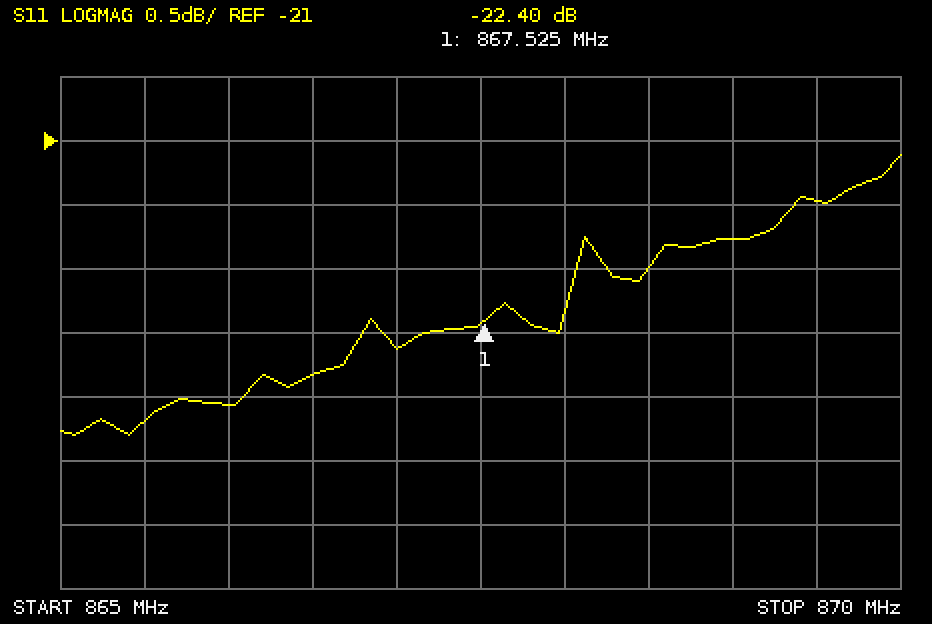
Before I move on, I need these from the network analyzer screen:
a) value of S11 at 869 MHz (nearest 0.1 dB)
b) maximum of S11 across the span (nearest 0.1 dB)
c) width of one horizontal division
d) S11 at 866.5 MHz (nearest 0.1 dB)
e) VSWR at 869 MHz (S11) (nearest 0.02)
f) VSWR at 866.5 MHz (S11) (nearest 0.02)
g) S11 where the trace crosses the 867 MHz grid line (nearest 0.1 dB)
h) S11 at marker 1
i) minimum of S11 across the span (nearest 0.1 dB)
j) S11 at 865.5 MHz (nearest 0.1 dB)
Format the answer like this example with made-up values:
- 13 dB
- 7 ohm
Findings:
- -21.8 dB
- -21.1 dB
- 500 kHz
- -22.8 dB
- 1.18
- 1.16
- -22.6 dB
- -22.40 dB
- -23.3 dB
- -23.2 dB
